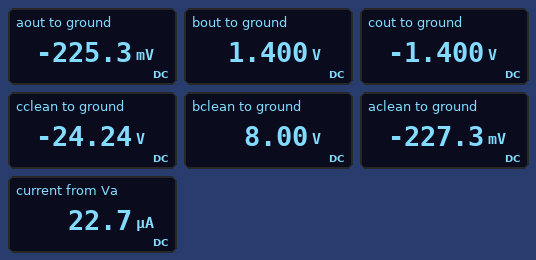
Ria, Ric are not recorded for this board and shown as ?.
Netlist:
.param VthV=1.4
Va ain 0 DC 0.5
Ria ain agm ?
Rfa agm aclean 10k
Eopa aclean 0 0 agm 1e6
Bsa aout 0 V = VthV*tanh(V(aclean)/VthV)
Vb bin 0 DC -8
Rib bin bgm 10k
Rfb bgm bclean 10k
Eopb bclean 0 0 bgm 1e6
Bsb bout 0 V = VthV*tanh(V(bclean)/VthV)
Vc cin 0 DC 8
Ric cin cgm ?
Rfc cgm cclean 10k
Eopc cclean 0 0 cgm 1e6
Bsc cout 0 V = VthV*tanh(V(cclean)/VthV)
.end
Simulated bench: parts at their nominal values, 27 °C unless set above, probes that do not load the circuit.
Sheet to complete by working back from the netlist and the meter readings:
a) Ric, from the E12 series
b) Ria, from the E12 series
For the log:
3.3 kΩ
22 kΩ
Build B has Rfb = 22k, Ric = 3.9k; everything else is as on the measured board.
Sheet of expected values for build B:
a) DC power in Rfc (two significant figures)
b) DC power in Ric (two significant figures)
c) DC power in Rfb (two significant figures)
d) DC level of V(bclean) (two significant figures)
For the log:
42 mW
16 mW
14 mW
18 V
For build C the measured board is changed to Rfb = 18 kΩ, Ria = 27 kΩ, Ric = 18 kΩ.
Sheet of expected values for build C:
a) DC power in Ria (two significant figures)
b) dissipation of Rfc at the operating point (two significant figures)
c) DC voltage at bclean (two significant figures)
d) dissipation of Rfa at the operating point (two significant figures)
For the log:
9.3 µW
2.0 mW
14 V
3.4 µW
